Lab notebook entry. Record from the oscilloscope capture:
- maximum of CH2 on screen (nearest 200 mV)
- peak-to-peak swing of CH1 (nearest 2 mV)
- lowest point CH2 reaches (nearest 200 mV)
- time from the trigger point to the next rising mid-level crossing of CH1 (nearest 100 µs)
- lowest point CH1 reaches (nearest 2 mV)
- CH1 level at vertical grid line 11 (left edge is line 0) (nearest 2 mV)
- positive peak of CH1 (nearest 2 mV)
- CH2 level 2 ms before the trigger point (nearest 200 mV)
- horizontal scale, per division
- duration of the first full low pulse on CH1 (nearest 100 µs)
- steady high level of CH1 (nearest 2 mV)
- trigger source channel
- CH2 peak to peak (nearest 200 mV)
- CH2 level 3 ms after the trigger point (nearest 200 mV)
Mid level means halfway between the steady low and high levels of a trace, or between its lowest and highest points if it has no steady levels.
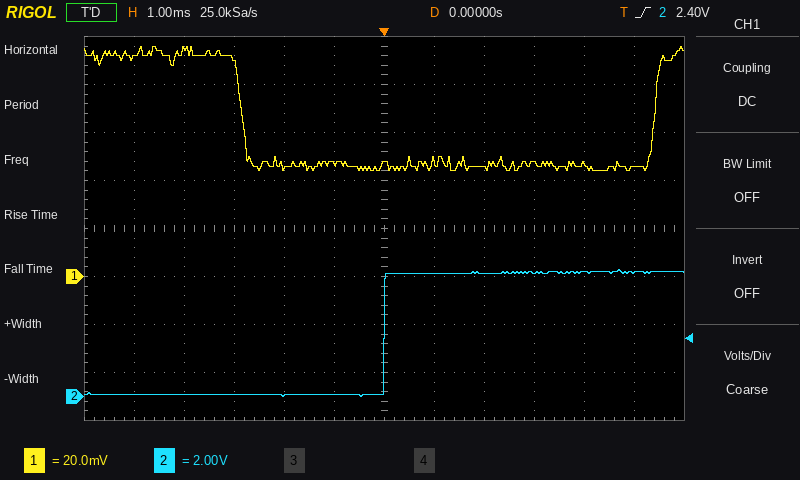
5.2 V
52 mV
0.0 V
5.4 ms
44 mV
46 mV
96 mV
0.0 V
1 ms
8.3 ms
92 mV
CH2
5.2 V
5.2 V
